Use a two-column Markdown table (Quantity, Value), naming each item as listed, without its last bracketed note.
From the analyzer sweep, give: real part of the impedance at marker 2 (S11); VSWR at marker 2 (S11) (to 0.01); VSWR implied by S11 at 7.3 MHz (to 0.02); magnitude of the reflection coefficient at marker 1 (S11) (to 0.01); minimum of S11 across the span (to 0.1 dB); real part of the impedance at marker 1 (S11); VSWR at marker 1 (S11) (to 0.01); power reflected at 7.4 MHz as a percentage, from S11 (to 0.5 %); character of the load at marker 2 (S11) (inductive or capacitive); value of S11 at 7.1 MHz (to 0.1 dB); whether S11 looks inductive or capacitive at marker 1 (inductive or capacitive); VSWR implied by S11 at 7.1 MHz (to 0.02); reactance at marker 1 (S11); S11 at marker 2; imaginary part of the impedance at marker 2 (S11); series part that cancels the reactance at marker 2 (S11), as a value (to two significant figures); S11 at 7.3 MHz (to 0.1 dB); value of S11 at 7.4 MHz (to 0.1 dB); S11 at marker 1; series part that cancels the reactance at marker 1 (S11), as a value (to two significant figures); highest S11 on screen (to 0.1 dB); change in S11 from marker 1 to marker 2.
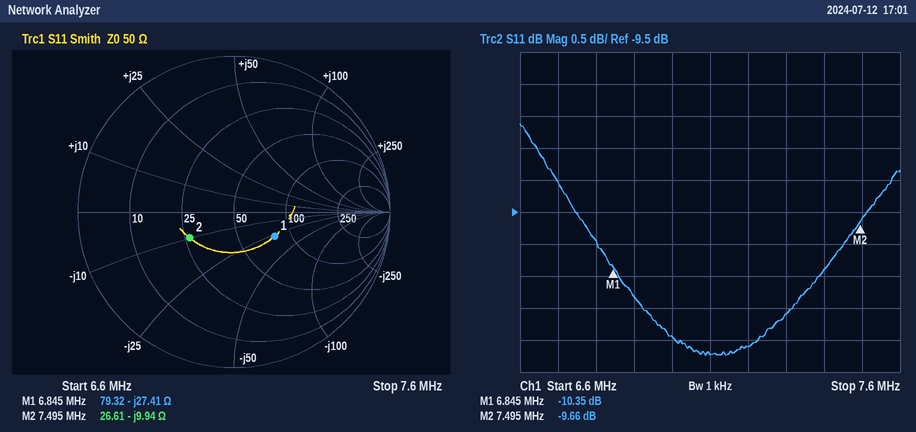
| Quantity | Value |
|---|---|
| real part of the impedance at marker 2 | 26.61 Ω |
| VSWR at marker 2 (S11) | 1.98 |
| VSWR implied by S11 at 7.3 MHz | 1.78 |
| magnitude of the reflection coefficient at marker 1 (S11) | 0.30 |
| minimum of S11 across the span | -11.7 dB |
| real part of the impedance at marker 1 | 79.32 Ω |
| VSWR at marker 1 (S11) | 1.87 |
| power reflected at 7.4 MHz as a percentage, from S11 | 9.0 % |
| character of the load at marker 2 (S11) | capacitive |
| value of S11 at 7.1 MHz | -11.7 dB |
| whether S11 looks inductive or capacitive at marker 1 | capacitive |
| VSWR implied by S11 at 7.1 MHz | 1.70 |
| reactance at marker 1 | -27.41 Ω |
| S11 at marker 2 | -9.66 dB |
| imaginary part of the impedance at marker 2 | -9.94 Ω |
| series part that cancels the reactance at marker 2 (S11), as a value | 210 nH |
| S11 at 7.3 MHz | -11.1 dB |
| value of S11 at 7.4 MHz | -10.4 dB |
| S11 at marker 1 | -10.35 dB |
| series part that cancels the reactance at marker 1 (S11), as a value | 640 nH |
| highest S11 on screen | -8.1 dB |
| change in S11 from marker 1 to marker 2 | 0.69 dB |
